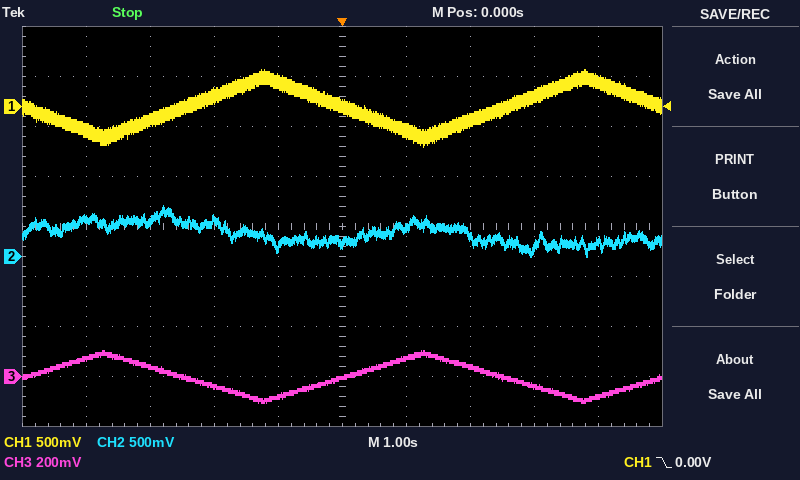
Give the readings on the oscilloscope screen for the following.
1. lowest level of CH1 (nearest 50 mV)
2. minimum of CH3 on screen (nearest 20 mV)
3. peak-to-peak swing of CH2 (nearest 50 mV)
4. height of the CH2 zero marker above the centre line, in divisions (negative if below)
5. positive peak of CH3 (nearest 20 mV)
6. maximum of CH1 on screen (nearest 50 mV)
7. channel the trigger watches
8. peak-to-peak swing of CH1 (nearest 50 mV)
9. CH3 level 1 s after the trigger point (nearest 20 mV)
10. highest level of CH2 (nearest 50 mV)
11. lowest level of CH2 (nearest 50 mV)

-400 mV
-100 mV
500 mV
-0.6 div
100 mV
350 mV
CH1
750 mV
80 mV
500 mV
0 mV
